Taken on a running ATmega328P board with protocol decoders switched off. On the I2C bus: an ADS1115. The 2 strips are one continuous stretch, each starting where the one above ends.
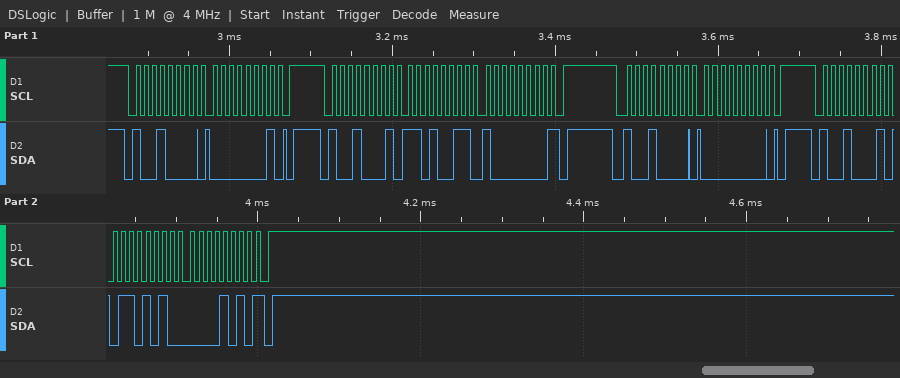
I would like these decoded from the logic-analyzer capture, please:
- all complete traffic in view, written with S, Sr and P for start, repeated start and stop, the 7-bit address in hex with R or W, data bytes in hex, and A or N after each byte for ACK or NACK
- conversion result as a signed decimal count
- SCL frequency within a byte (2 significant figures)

S 48W A 01 A P S 48R A D3 A 80 N P S 48W A 00 A P S 48R A 6A A 0A N P
27146
100 kHz
